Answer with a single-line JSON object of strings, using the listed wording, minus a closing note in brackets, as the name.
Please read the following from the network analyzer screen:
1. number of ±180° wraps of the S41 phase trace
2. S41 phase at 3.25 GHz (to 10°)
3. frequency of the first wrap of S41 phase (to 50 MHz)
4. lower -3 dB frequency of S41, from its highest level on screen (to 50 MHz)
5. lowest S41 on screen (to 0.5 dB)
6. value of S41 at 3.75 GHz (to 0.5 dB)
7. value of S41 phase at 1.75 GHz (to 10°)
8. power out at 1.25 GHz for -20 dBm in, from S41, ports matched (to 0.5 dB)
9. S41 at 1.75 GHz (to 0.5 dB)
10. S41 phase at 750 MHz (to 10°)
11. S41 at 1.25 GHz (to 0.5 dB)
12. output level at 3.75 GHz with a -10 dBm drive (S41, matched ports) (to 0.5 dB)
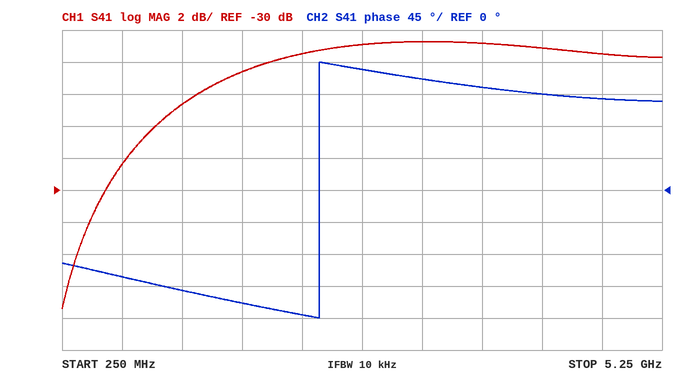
{"number of ±180° wraps of the S41 phase trace": "1", "S41 phase at 3.25 GHz": "160°", "frequency of the first wrap of S41 phase": "2.40 GHz", "lower -3 dB frequency of S41, from its highest level on screen": "1.45 GHz", "lowest S41 on screen": "-37.5 dB", "value of S41 at 3.75 GHz": "-21.0 dB", "value of S41 phase at 1.75 GHz": "-160°", "power out at 1.25 GHz for -20 dBm in, from S41, ports matched": "-44.5 dBm", "S41 at 1.75 GHz": "-22.5 dB", "S41 phase at 750 MHz": "-120°", "S41 at 1.25 GHz": "-24.5 dB", "output level at 3.75 GHz with a -10 dBm drive (S41, matched ports)": "-31.0 dBm"}
